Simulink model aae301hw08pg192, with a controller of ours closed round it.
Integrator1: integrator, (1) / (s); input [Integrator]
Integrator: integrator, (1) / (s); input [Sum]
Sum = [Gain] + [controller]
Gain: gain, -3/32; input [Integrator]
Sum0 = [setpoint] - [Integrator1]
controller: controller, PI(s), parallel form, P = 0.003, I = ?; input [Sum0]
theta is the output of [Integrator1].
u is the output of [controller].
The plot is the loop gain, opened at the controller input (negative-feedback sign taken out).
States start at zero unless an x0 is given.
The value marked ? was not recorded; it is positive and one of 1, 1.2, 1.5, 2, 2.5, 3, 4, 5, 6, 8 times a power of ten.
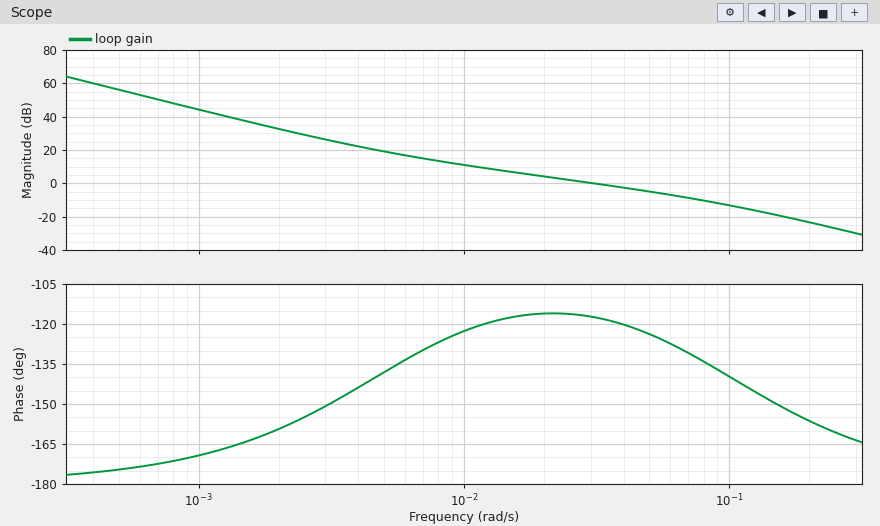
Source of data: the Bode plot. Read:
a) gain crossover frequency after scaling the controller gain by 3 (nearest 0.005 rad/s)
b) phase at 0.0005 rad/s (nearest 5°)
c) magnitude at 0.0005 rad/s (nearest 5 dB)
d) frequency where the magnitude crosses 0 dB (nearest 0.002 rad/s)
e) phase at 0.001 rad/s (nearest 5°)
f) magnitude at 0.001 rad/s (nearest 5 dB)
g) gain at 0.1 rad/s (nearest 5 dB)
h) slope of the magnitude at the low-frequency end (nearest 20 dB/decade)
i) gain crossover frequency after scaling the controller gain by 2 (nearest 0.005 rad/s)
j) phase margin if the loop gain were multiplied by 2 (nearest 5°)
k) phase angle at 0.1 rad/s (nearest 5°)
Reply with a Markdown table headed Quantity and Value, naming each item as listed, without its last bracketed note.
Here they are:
| Quantity | Value |
|---|---|
| gain crossover frequency after scaling the controller gain by 3 | 0.075 rad/s |
| phase at 0.0005 rad/s | -175° |
| magnitude at 0.0005 rad/s | 55 dB |
| frequency where the magnitude crosses 0 dB | 0.030 rad/s |
| phase at 0.001 rad/s | -170° |
| magnitude at 0.001 rad/s | 45 dB |
| gain at 0.1 rad/s | -15 dB |
| slope of the magnitude at the low-frequency end | -40 dB/decade |
| gain crossover frequency after scaling the controller gain by 2 | 0.055 rad/s |
| phase margin if the loop gain were multiplied by 2 | 55° |
| phase angle at 0.1 rad/s | -140° |
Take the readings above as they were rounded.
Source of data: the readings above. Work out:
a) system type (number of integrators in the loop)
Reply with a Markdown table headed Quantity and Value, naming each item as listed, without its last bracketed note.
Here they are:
| Quantity | Value |
|---|---|
| system type | 2 |
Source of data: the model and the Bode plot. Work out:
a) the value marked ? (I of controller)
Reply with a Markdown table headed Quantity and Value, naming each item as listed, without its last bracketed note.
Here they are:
| Quantity | Value |
|---|---|
| the value marked ? | 1.5e-05 |
